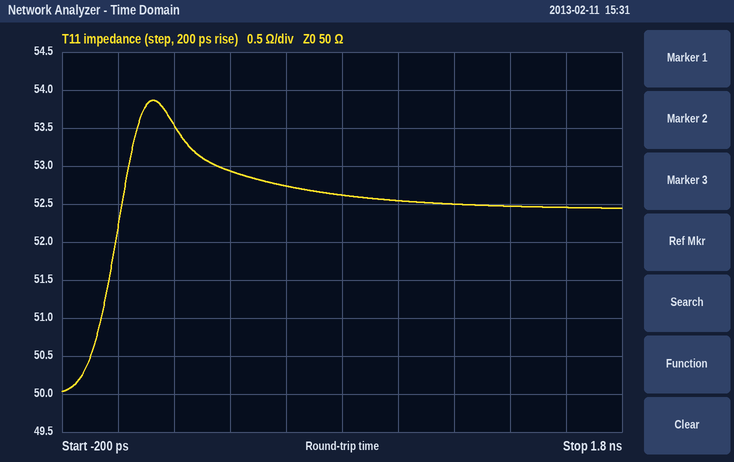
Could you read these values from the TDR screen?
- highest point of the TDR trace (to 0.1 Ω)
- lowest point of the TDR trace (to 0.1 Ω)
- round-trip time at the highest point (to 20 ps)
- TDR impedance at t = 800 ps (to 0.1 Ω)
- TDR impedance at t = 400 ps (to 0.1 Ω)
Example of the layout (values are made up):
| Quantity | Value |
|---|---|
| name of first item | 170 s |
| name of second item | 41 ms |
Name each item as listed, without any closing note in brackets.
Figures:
| Quantity | Value |
|---|---|
| highest point of the TDR trace | 53.9 Ω |
| lowest point of the TDR trace | 50.0 Ω |
| round-trip time at the highest point | 120 ps |
| TDR impedance at t = 800 ps | 52.6 Ω |
| TDR impedance at t = 400 ps | 52.9 Ω |
